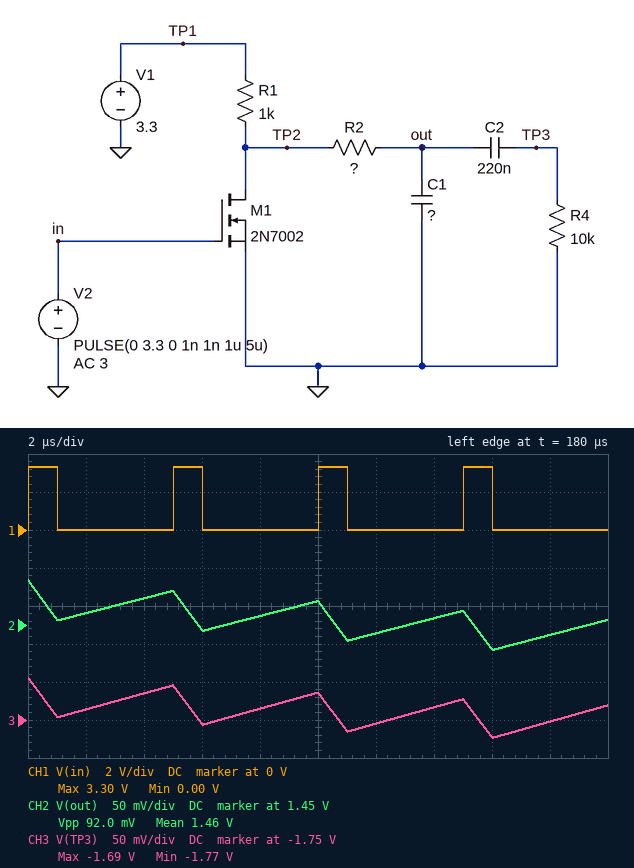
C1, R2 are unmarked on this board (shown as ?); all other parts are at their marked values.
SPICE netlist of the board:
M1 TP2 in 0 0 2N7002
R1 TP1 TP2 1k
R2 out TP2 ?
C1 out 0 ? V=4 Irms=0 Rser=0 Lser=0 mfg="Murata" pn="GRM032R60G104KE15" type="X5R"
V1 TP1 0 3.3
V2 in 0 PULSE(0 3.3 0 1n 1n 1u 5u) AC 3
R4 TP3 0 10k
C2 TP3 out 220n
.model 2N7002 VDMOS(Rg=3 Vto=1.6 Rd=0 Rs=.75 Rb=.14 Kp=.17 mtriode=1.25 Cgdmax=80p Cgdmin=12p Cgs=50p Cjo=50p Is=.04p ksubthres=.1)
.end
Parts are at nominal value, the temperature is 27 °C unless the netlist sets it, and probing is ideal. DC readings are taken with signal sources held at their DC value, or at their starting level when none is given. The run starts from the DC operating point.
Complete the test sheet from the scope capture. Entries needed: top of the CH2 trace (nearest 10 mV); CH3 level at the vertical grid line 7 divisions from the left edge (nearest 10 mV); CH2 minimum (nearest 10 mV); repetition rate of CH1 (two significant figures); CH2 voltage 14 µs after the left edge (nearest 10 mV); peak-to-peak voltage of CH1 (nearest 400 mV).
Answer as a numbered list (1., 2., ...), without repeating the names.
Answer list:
1. 1.51 V
2. -1.73 V
3. 1.42 V
4. 200 kHz
5. 1.46 V
6. 3.2 V
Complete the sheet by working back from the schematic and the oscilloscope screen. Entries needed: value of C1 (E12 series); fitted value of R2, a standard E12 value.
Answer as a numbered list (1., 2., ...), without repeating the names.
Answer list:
1. 180 nF
2. 150 Ω
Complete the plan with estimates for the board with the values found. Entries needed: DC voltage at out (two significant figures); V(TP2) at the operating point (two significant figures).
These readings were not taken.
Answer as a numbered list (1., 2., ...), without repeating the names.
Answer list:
1. 3.3 V
2. 3.3 V
